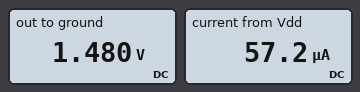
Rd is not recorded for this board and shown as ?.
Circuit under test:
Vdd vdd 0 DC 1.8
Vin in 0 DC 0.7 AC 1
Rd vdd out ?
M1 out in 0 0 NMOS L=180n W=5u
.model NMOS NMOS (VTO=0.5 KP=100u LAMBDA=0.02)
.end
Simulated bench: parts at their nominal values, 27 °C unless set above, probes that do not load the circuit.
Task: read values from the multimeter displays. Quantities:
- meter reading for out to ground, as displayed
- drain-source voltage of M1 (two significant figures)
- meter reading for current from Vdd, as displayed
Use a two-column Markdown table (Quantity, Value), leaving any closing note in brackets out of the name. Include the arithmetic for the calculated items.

| Quantity | Value |
|---|---|
| meter reading for out to ground, as displayed | 1.480 V |
| drain-source voltage of M1 | 1.48 V = 1.5 V |
| meter reading for current from Vdd, as displayed | 57.2 µA |
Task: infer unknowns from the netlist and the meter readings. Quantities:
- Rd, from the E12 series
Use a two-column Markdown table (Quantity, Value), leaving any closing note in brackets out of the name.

| Quantity | Value |
|---|---|
| Rd, from the E12 series | 5.6 kΩ |
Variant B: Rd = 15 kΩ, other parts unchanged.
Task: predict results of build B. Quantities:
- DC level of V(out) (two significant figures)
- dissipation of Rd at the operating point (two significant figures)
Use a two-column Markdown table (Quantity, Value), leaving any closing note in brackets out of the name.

| Quantity | Value |
|---|---|
| DC level of V(out) | 950 mV |
| dissipation of Rd at the operating point | 48 µW |
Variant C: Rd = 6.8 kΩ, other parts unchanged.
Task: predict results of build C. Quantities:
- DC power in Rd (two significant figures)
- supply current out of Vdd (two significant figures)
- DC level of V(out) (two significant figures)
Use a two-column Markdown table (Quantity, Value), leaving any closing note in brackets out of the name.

| Quantity | Value |
|---|---|
| DC power in Rd | 22 µW |
| supply current out of Vdd | 57 µA |
| DC level of V(out) | 1.4 V |
